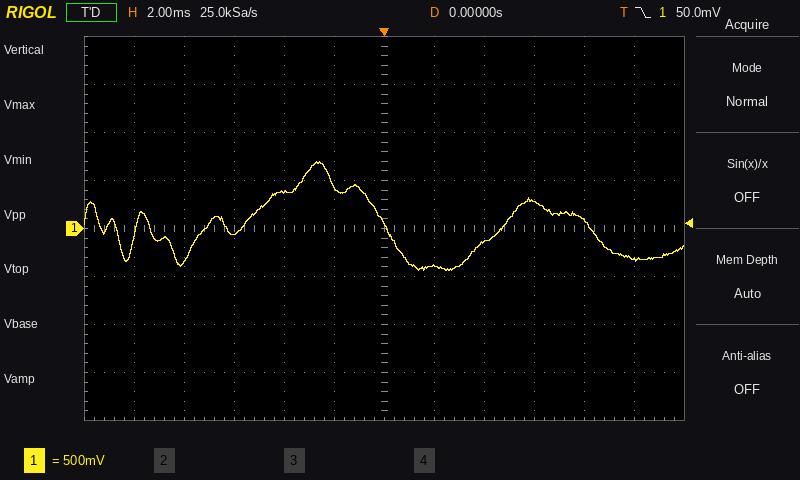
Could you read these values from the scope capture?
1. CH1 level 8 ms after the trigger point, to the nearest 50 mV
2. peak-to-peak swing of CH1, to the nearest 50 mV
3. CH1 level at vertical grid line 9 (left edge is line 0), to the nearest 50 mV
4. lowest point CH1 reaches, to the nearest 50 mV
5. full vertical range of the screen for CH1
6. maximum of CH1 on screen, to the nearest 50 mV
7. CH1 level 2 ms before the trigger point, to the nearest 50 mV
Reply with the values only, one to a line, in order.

100 mV
1.15 V
300 mV
-450 mV
4 V
700 mV
450 mV
